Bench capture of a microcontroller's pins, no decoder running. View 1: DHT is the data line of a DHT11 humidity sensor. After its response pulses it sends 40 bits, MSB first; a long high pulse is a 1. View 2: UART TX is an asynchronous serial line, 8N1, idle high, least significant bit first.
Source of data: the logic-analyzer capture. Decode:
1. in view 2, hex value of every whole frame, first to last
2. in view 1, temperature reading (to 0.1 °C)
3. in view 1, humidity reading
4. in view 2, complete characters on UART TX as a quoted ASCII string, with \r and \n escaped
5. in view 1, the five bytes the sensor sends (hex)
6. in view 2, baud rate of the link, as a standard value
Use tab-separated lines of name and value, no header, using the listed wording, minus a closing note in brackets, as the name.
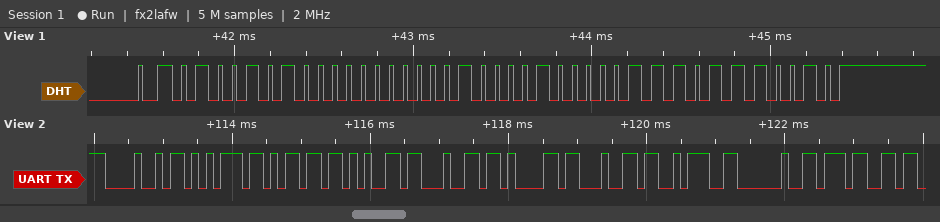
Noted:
in view 2, hex value of every whole frame, first to last	48 75 6D 65 64 61 64 3A 20 37
in view 1, temperature reading	33.7 °C
in view 1, humidity reading	74 %
in view 2, complete characters on UART TX as a quoted ASCII string, with \r and \n escaped	"Humedad: 7"
in view 1, the five bytes the sensor sends	4A 00 21 07 72
in view 2, baud rate of the link, as a standard value	9600 baud
